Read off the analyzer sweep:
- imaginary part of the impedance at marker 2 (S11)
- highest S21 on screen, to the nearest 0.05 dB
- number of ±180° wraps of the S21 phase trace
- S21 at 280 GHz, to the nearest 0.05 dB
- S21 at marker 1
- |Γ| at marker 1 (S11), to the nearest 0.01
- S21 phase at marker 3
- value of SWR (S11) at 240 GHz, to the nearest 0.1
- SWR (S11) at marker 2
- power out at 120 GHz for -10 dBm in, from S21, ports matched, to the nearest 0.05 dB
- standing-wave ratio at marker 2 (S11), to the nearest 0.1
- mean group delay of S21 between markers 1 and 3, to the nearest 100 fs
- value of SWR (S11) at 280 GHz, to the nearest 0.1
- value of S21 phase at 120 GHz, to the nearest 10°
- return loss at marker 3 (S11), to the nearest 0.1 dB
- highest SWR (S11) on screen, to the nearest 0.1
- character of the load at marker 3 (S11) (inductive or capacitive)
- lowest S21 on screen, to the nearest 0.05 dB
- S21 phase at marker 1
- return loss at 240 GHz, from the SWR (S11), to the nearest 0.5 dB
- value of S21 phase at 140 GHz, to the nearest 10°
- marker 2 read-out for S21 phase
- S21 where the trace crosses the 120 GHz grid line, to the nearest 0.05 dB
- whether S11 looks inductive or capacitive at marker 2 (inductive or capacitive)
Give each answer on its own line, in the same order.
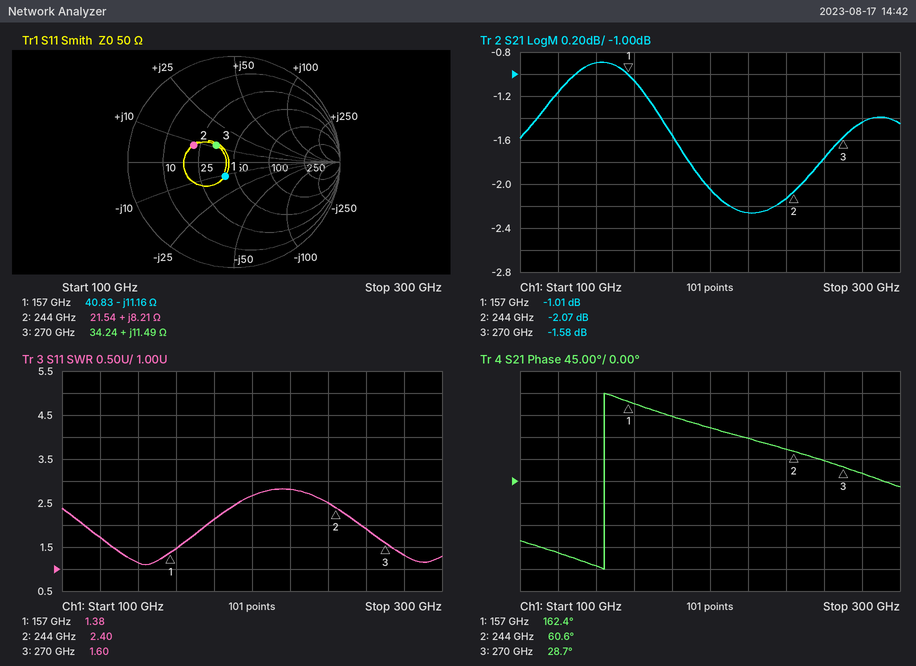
+8.21 Ω
-0.90 dB
1
-1.45 dB
-1.01 dB
0.16
28.7°
2.5
2.40
-11.15 dBm
2.4
3.3 ps
1.3
-150°
12.8 dB
2.8
inductive
-2.25 dB
162.4°
7.5 dB
-170°
60.6°
-1.15 dB
inductive
